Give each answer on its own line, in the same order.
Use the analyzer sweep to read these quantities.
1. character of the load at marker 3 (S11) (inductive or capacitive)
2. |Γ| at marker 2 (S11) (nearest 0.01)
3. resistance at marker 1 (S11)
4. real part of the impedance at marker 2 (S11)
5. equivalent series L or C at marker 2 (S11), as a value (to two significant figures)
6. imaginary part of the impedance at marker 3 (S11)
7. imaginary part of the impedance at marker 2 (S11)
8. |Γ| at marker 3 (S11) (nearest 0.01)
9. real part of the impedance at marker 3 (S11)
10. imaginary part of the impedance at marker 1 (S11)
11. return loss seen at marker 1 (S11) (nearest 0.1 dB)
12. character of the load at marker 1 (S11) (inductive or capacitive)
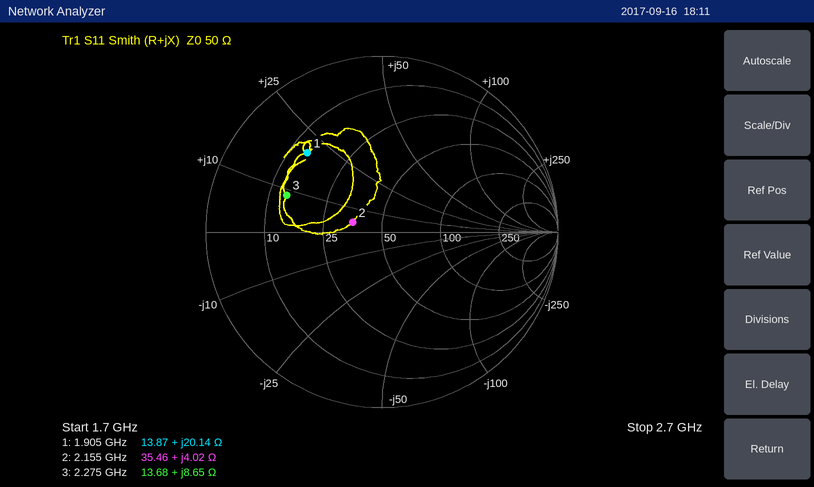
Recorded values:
inductive
0.18
13.87 Ω
35.46 Ω
300 pH
+8.65 Ω
+4.02 Ω
0.58
13.68 Ω
+20.14 Ω
4.2 dB
inductive
